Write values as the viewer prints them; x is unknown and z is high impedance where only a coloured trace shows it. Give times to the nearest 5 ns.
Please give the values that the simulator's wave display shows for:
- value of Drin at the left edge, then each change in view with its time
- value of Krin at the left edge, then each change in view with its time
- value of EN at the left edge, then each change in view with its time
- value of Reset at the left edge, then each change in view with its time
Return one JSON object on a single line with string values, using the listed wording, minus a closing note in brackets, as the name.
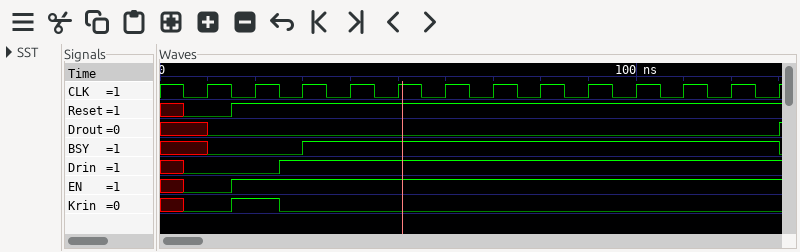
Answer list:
{"value of Drin at the left edge, then each change in view with its time": "x, 0 at 5 ns, 1 at 25 ns", "value of Krin at the left edge, then each change in view with its time": "x, 0 at 5 ns, 1 at 15 ns, 0 at 25 ns", "value of EN at the left edge, then each change in view with its time": "x, 0 at 5 ns, 1 at 15 ns", "value of Reset at the left edge, then each change in view with its time": "x, 0 at 5 ns, 1 at 15 ns"}
